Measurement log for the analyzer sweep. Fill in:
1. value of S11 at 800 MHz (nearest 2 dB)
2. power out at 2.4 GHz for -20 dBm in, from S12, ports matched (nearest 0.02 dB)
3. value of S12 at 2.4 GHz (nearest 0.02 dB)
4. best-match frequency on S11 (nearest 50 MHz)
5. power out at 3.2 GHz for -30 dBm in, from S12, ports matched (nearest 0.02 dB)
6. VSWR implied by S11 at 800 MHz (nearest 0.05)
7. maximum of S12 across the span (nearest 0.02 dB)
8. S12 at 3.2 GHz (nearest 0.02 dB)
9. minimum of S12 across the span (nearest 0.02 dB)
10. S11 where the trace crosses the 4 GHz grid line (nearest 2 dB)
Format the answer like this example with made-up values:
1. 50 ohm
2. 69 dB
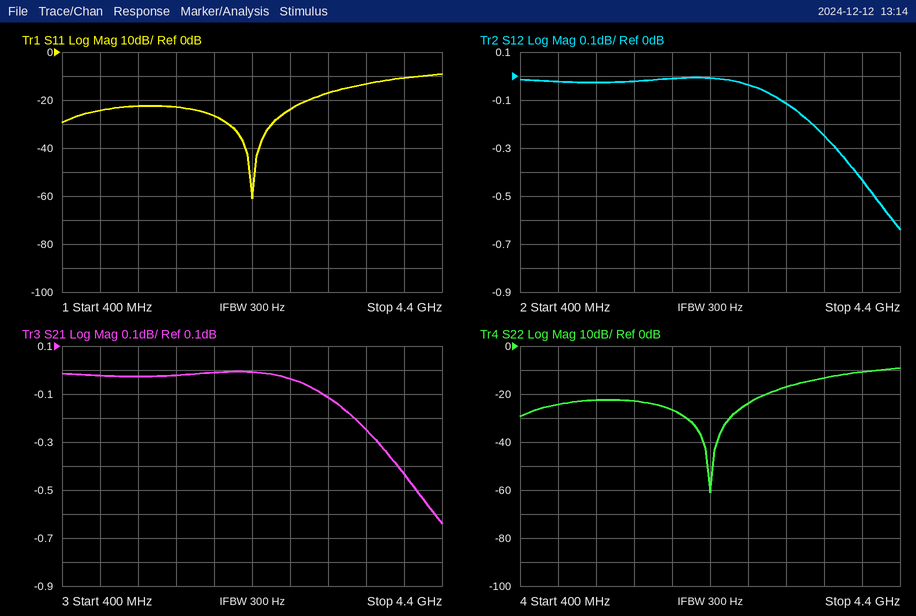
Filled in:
1. -24 dB
2. -20.00 dBm
3. 0.00 dB
4. 2.40 GHz
5. -30.12 dBm
6. 1.15
7. 0.00 dB
8. -0.12 dB
9. -0.64 dB
10. -10 dB
